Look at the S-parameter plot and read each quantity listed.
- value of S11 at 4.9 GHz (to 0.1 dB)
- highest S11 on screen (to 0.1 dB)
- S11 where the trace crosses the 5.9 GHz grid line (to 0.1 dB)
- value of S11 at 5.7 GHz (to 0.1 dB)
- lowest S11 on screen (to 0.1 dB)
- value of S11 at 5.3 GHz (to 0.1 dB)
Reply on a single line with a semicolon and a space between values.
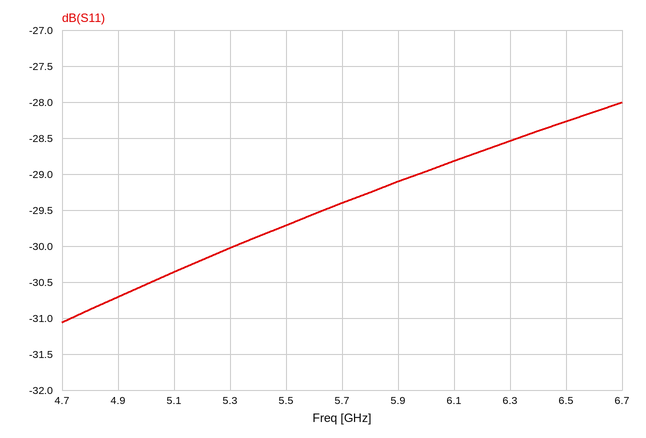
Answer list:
-30.7 dB; -28.0 dB; -29.1 dB; -29.4 dB; -31.1 dB; -30.0 dB
